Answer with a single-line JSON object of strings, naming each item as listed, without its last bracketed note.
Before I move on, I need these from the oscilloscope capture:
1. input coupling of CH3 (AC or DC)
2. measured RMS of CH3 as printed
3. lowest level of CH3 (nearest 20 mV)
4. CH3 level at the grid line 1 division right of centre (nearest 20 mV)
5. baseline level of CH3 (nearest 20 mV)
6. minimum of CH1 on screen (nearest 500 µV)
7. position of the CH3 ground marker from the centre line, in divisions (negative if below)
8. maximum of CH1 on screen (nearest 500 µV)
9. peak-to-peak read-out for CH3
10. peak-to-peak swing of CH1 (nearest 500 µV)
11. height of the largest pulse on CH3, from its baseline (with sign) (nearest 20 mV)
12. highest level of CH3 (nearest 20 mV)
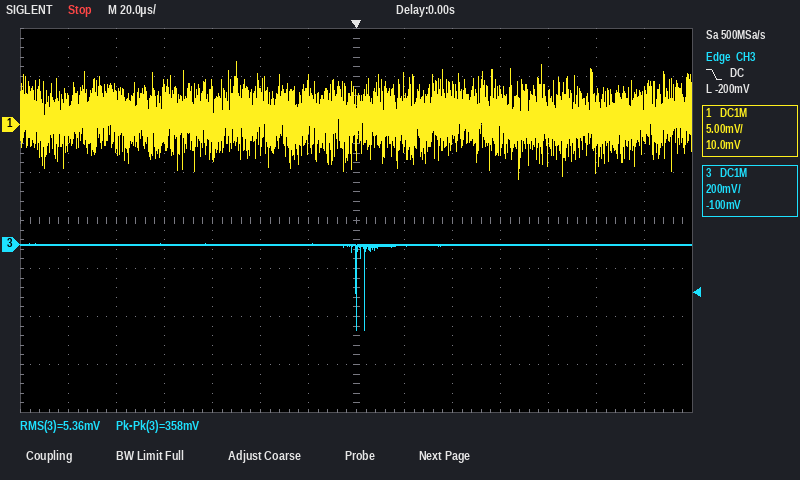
{"input coupling of CH3": "DC", "measured RMS of CH3 as printed": "5.36 mV", "lowest level of CH3": "-360 mV", "CH3 level at the grid line 1 division right of centre": "0 mV", "baseline level of CH3": "0 mV", "minimum of CH1 on screen": "-5.5 mV", "position of the CH3 ground marker from the centre line, in divisions": "-0.5 div", "maximum of CH1 on screen": "6.5 mV", "peak-to-peak read-out for CH3": "358 mV", "peak-to-peak swing of CH1": "12.0 mV", "height of the largest pulse on CH3, from its baseline (with sign)": "-360 mV", "highest level of CH3": "0 mV"}
